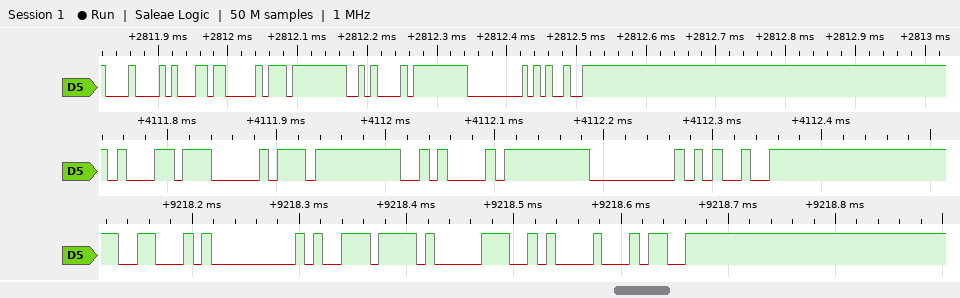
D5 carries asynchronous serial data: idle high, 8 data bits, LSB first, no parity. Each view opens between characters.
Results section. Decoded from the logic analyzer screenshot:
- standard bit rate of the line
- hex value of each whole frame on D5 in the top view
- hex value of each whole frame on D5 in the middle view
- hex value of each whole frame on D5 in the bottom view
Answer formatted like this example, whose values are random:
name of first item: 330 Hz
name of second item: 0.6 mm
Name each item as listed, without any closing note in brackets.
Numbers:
standard bit rate of the line: 115200 baud
hex value of each whole frame on D5 in the top view: 08, B1, D0, FF, 0A, FF, 00, 25
hex value of each whole frame on D5 in the middle view: B1, D0, FF, 0A, FF, 00, 25
hex value of each whole frame on D5 in the bottom view: 46, 00, B9, C1, 0A, 34
